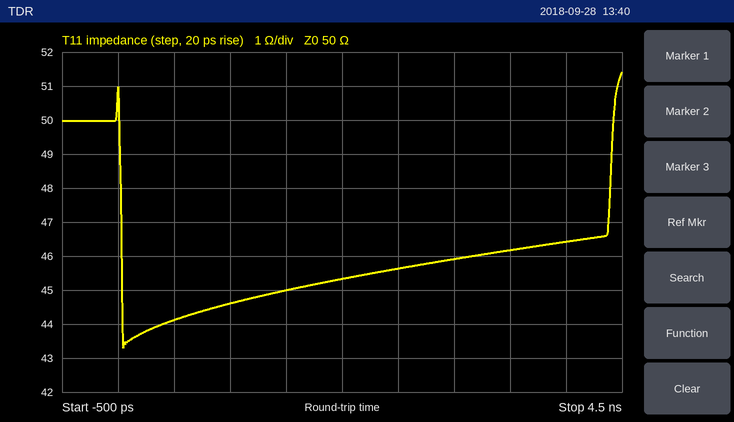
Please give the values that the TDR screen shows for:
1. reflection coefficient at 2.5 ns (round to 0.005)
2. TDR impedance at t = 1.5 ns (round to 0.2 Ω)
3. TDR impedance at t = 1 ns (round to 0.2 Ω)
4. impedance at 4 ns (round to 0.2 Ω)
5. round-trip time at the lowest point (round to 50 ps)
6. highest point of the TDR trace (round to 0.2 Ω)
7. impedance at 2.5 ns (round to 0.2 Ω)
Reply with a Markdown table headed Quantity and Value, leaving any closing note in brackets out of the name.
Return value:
| Quantity | Value |
|---|---|
| reflection coefficient at 2.5 ns | -0.045 |
| TDR impedance at t = 1.5 ns | 45.0 Ω |
| TDR impedance at t = 1 ns | 44.6 Ω |
| impedance at 4 ns | 46.4 Ω |
| round-trip time at the lowest point | 50 ps |
| highest point of the TDR trace | 51.4 Ω |
| impedance at 2.5 ns | 45.6 Ω |
